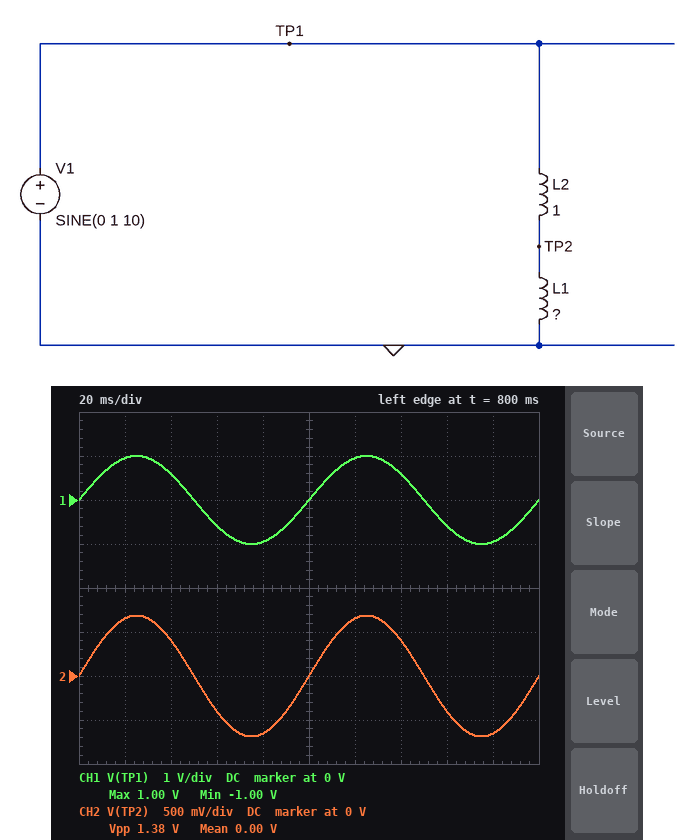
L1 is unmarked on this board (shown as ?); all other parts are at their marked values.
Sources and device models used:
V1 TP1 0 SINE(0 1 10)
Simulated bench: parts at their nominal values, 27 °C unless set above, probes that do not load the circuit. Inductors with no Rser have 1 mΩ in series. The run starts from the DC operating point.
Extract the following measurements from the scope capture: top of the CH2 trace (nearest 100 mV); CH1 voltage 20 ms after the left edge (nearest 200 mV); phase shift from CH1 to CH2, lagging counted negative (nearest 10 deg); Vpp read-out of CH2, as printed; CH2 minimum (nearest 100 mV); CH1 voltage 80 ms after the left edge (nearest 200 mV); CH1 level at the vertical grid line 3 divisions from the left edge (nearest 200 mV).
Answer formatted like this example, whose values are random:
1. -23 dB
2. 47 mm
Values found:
1. 700 mV
2. 1.0 V
3. 0 deg
4. 1.38 V
5. -700 mV
6. -1.0 V
7. -600 mV
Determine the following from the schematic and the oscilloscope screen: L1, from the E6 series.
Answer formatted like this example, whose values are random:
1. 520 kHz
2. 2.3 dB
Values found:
1. 2.2 H
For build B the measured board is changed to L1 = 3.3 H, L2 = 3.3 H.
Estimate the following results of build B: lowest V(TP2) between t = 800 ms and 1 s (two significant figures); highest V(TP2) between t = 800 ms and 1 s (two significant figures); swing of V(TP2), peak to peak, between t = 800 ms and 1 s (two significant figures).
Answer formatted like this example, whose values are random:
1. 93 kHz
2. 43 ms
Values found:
1. -500 mV
2. 500 mV
3. 1.0 V
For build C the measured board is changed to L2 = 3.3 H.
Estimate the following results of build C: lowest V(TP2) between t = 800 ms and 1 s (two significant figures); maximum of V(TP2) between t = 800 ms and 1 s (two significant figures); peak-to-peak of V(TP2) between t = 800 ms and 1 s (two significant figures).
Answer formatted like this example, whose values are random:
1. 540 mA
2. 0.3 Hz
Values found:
1. -400 mV
2. 400 mV
3. 800 mV
